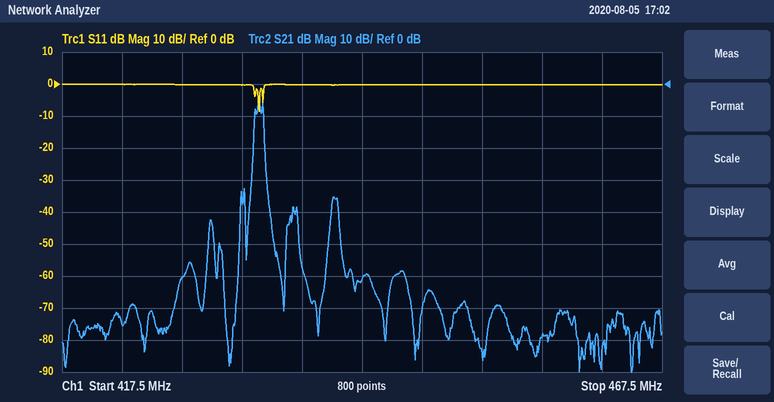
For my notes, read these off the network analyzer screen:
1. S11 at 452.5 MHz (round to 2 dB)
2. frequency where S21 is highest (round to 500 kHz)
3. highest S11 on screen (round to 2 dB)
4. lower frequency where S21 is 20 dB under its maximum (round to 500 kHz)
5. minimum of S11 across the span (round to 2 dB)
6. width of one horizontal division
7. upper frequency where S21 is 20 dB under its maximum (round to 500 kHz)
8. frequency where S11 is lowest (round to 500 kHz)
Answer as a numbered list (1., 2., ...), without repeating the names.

1. 0 dB
2. 434.0 MHz
3. 0 dB
4. 433.5 MHz
5. -8 dB
6. 5 MHz
7. 434.5 MHz
8. 434.0 MHz
